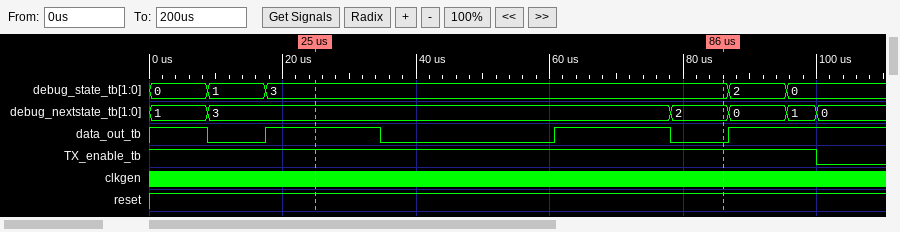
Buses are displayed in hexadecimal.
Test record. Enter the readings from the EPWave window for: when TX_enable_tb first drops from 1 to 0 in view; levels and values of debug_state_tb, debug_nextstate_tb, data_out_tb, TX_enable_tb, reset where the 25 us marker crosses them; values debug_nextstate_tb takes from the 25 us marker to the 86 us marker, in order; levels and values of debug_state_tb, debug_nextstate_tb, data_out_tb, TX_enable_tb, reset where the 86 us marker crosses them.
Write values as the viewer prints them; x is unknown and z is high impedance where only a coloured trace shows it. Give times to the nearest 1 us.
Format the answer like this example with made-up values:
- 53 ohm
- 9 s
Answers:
- 100 us
- debug_state_tb=3, debug_nextstate_tb=3, data_out_tb=1, TX_enable_tb=1, reset=1
- 3, 2
- debug_state_tb=3, debug_nextstate_tb=2, data_out_tb=0, TX_enable_tb=1, reset=1
